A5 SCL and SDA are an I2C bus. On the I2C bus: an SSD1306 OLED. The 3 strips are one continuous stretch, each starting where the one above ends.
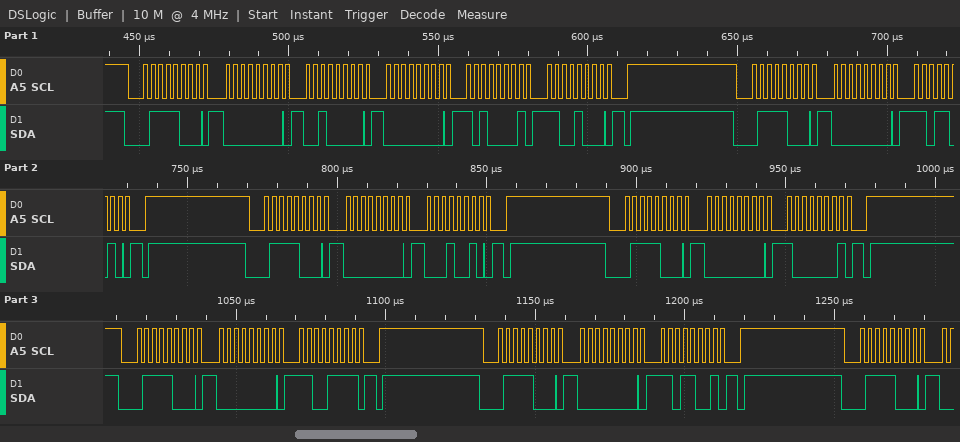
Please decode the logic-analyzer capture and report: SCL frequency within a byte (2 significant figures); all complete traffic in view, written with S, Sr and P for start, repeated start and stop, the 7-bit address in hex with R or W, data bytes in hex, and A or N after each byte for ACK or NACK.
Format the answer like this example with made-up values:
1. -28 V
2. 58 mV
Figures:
1. 400 kHz
2. S 3CW A 00 A 20 A 00 A A1 A C8 A P S 3CW A 00 A DA A P S 3CW A 00 A 12 A P S 3CW A 00 A 81 A P S 3CW A 00 A CF A P S 3CW A 00 A D9 A P S 3CW A
